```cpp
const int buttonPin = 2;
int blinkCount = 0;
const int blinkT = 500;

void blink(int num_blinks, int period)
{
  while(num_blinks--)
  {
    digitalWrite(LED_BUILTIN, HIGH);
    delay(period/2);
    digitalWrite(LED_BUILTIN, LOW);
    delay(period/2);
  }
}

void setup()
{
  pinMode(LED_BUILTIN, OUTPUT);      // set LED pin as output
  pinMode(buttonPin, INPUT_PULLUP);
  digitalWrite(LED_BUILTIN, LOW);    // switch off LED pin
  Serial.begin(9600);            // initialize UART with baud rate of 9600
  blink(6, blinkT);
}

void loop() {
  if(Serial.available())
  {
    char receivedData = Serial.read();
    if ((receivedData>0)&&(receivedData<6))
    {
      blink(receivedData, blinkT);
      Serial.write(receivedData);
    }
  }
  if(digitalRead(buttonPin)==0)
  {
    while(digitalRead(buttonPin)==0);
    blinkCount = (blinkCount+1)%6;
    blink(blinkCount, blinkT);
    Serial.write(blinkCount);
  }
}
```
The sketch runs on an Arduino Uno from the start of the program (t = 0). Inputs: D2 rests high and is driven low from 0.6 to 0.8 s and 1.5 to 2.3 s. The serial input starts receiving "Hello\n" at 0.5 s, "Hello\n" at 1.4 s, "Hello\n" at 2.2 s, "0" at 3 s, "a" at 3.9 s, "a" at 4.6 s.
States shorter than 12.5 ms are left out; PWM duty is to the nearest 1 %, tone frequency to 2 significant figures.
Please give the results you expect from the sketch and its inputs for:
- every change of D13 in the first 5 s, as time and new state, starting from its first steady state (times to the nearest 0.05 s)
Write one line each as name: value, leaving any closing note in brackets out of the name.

every change of D13 in the first 5 s, as time and new state, starting from its first steady state: 0 s high; 0.25 s low; 0.5 s high; 0.75 s low; 1 s high; 1.25 s low; 1.5 s high; 1.75 s low; 2 s high; 2.25 s low; 2.5 s high; 2.75 s low
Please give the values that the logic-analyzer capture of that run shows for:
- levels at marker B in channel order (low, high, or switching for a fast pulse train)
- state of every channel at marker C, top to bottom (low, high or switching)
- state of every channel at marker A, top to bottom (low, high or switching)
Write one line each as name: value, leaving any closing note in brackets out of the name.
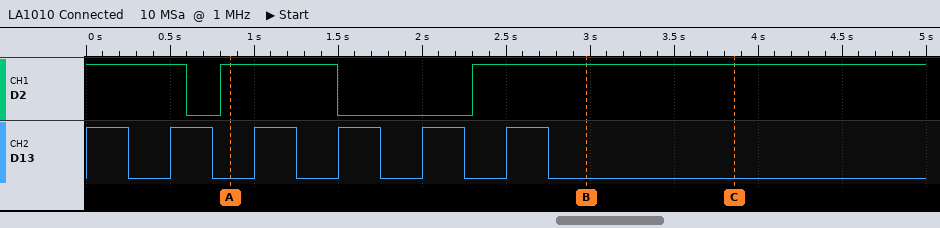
levels at marker B in channel order: D2 high, D13 low
state of every channel at marker C, top to bottom: D2 high, D13 low
state of every channel at marker A, top to bottom: D2 high, D13 low
